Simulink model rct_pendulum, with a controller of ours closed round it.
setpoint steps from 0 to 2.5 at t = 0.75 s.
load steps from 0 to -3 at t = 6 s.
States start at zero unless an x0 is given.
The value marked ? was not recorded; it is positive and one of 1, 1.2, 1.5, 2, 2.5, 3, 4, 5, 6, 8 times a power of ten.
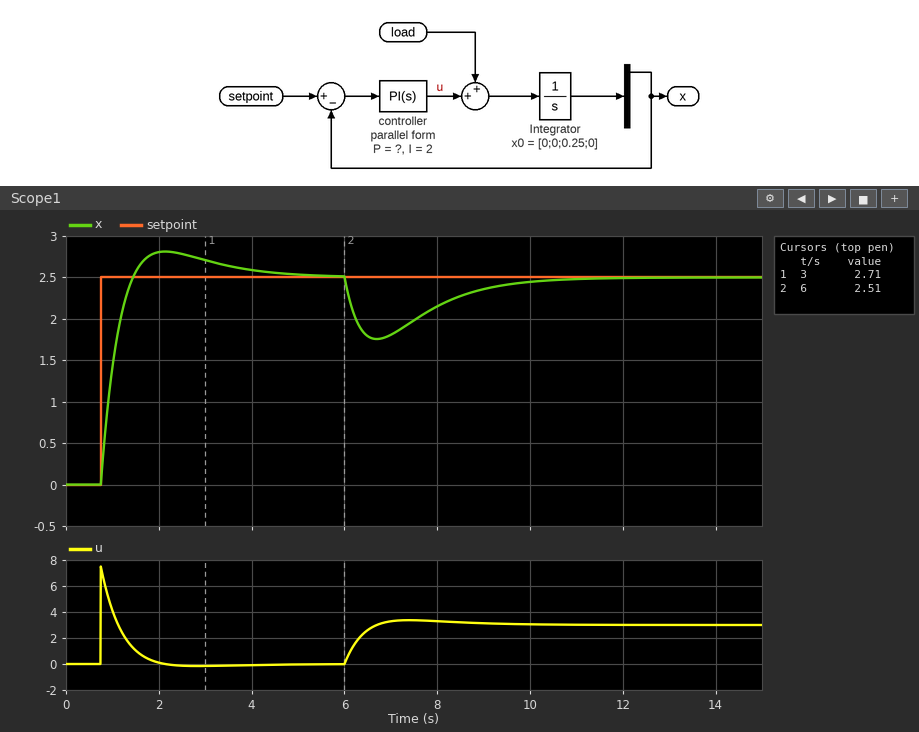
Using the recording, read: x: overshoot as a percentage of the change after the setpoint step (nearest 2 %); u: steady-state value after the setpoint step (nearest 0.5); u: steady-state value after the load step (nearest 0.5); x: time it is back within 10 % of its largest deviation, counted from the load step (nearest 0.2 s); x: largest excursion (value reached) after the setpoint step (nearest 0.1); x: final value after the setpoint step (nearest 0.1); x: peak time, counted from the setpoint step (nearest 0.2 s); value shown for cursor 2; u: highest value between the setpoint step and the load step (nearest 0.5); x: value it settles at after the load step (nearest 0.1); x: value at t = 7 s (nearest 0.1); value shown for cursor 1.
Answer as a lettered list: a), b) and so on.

a) 12 %
b) 0.0
c) 3.0
d) 3.6 s
e) 2.8
f) 2.5
g) 1.4 s
h) 2.51
i) 7.5
j) 2.5
k) 1.8
l) 2.71
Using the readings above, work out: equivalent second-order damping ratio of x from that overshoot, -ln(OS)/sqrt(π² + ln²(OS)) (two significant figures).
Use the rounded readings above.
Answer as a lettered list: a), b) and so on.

a) 0.56
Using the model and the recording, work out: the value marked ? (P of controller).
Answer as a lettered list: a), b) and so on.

a) 3
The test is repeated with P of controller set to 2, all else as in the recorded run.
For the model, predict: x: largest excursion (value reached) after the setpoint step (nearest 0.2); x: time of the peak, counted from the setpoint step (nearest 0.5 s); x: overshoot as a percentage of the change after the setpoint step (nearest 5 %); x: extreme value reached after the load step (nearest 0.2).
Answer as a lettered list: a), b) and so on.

a) 3.0
b) 1.5 s
c) 20 %
d) 1.6
